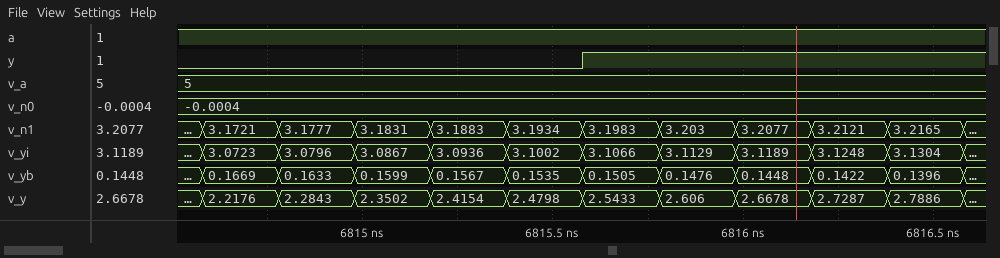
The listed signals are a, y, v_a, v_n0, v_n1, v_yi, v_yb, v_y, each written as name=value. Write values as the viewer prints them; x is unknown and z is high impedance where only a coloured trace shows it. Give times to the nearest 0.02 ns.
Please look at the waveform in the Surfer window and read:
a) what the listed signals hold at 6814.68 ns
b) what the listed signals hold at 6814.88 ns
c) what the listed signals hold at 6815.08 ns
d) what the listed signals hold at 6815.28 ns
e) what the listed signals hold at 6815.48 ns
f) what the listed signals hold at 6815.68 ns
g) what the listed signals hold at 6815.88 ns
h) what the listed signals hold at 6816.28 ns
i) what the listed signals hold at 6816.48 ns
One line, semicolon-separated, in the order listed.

a=1, y=0, v_a=5, v_n0=-0.0004, v_n1=3.1721, v_yi=3.0723, v_yb=0.1669, v_y=2.2176; a=1, y=0, v_a=5, v_n0=-0.0004, v_n1=3.1777, v_yi=3.0796, v_yb=0.1633, v_y=2.2843; a=1, y=0, v_a=5, v_n0=-0.0004, v_n1=3.1831, v_yi=3.0867, v_yb=0.1599, v_y=2.3502; a=1, y=0, v_a=5, v_n0=-0.0004, v_n1=3.1883, v_yi=3.0936, v_yb=0.1567, v_y=2.4154; a=1, y=0, v_a=5, v_n0=-0.0004, v_n1=3.1934, v_yi=3.1002, v_yb=0.1535, v_y=2.4798; a=1, y=1, v_a=5, v_n0=-0.0004, v_n1=3.1983, v_yi=3.1066, v_yb=0.1505, v_y=2.5433; a=1, y=1, v_a=5, v_n0=-0.0004, v_n1=3.203, v_yi=3.1129, v_yb=0.1476, v_y=2.606; a=1, y=1, v_a=5, v_n0=-0.0004, v_n1=3.2121, v_yi=3.1248, v_yb=0.1422, v_y=2.7287; a=1, y=1, v_a=5, v_n0=-0.0004, v_n1=3.2165, v_yi=3.1304, v_yb=0.1396, v_y=2.7886
